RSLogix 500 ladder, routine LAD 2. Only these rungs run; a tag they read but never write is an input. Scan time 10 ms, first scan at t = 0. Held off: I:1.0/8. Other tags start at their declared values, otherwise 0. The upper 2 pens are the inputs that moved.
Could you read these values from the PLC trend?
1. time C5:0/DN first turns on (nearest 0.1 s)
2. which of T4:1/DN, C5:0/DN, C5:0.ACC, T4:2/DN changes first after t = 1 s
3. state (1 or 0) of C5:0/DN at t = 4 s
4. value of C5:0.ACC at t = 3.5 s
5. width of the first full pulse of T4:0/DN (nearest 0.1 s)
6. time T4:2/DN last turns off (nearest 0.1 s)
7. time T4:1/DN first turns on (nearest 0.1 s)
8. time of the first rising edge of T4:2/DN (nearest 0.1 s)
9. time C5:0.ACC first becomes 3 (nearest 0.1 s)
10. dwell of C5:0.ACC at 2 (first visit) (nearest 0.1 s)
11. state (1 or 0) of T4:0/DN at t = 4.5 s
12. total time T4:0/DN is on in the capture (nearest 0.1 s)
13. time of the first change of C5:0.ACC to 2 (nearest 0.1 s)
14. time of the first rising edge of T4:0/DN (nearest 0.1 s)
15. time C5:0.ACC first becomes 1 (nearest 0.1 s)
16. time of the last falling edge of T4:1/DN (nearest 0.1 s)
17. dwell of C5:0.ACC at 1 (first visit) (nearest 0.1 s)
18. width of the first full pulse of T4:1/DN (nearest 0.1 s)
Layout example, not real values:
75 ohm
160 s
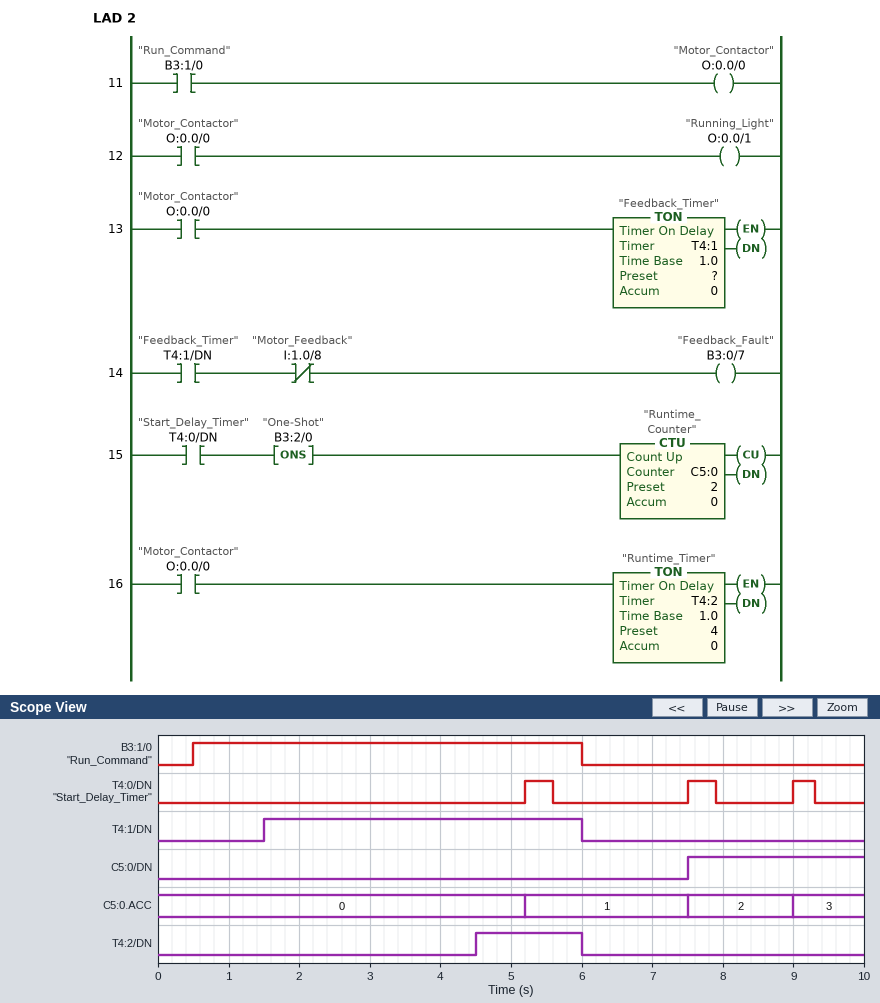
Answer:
7.5 s
T4:1/DN
0
0
0.4 s
6.0 s
1.5 s
4.5 s
9.0 s
1.5 s
0
1.1 s
7.5 s
5.2 s
5.2 s
6.0 s
2.3 s
4.5 s
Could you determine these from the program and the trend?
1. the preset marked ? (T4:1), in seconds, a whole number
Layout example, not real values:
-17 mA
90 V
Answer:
1 s
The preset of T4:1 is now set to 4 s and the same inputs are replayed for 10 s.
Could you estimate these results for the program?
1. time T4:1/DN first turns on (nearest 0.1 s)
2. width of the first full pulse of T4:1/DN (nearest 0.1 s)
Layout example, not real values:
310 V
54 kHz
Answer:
4.5 s
1.5 s
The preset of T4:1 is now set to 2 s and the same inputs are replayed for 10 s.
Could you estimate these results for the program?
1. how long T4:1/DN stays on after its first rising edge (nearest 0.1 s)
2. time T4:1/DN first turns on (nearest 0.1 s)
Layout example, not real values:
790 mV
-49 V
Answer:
3.5 s
2.5 s
